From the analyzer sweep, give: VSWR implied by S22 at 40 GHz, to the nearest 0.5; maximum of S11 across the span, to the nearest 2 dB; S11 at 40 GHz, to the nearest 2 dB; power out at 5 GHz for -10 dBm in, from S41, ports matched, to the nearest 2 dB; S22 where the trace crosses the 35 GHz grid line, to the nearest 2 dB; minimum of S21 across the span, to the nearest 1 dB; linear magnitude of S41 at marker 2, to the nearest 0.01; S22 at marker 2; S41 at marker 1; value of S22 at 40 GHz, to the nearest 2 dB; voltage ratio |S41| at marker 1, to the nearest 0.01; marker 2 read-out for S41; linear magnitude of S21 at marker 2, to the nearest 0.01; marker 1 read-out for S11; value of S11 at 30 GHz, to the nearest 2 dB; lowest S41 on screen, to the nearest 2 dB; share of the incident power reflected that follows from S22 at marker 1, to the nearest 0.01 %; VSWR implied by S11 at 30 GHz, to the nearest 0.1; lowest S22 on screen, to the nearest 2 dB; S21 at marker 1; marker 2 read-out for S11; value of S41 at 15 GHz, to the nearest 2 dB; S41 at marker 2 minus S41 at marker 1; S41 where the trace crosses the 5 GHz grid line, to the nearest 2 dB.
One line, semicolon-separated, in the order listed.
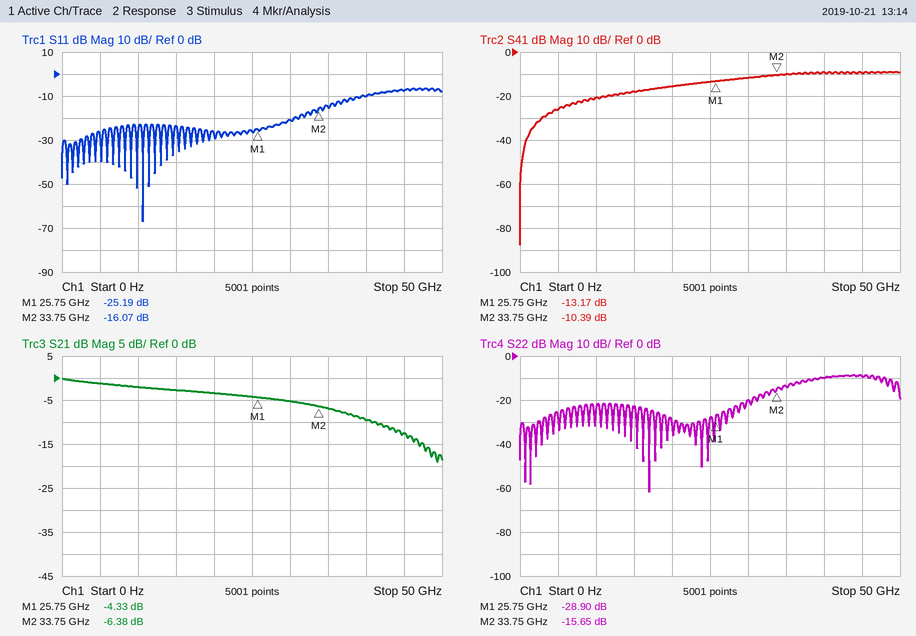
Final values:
2.0; -6 dB; -10 dB; -36 dBm; -14 dB; -19 dB; 0.30; -15.65 dB; -13.17 dB; -10 dB; 0.22; -10.39 dB; 0.48; -25.19 dB; -20 dB; -88 dB; 0.13 %; 1.2; -62 dB; -4.33 dB; -16.07 dB; -18 dB; 2.78 dB; -26 dB
